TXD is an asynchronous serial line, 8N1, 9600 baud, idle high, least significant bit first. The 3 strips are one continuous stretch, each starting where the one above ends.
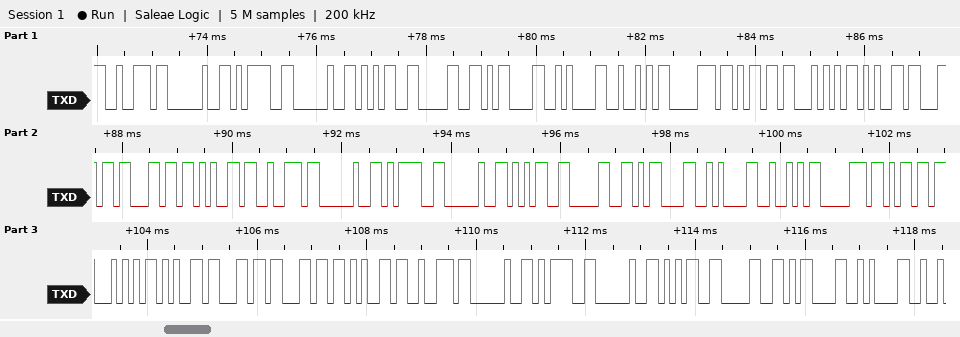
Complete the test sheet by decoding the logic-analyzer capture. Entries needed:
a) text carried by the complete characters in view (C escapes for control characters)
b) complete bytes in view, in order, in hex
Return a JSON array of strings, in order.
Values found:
["\"r = 50\\r\\nRpmTeller = 50\\r\\nRpmTeller = 50\\r\\n\"", "72 20 3D 20 35 30 0D 0A 52 70 6D 54 65 6C 6C 65 72 20 3D 20 35 30 0D 0A 52 70 6D 54 65 6C 6C 65 72 20 3D 20 35 30 0D 0A"]
